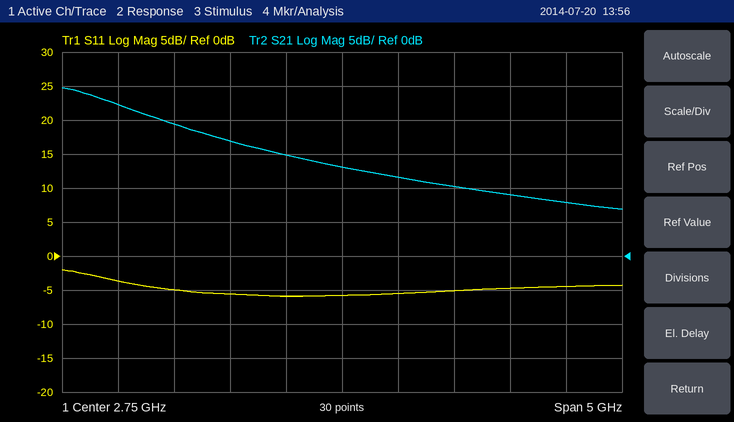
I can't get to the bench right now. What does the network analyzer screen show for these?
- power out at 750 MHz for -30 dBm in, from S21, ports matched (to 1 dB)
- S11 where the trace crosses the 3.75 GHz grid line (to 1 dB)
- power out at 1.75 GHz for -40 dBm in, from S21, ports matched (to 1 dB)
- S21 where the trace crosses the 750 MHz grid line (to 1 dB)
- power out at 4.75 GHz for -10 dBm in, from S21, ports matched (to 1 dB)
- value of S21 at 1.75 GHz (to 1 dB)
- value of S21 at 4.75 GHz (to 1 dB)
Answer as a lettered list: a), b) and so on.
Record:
a) -8 dBm
b) -5 dB
c) -23 dBm
d) 22 dB
e) -2 dBm
f) 17 dB
g) 8 dB
